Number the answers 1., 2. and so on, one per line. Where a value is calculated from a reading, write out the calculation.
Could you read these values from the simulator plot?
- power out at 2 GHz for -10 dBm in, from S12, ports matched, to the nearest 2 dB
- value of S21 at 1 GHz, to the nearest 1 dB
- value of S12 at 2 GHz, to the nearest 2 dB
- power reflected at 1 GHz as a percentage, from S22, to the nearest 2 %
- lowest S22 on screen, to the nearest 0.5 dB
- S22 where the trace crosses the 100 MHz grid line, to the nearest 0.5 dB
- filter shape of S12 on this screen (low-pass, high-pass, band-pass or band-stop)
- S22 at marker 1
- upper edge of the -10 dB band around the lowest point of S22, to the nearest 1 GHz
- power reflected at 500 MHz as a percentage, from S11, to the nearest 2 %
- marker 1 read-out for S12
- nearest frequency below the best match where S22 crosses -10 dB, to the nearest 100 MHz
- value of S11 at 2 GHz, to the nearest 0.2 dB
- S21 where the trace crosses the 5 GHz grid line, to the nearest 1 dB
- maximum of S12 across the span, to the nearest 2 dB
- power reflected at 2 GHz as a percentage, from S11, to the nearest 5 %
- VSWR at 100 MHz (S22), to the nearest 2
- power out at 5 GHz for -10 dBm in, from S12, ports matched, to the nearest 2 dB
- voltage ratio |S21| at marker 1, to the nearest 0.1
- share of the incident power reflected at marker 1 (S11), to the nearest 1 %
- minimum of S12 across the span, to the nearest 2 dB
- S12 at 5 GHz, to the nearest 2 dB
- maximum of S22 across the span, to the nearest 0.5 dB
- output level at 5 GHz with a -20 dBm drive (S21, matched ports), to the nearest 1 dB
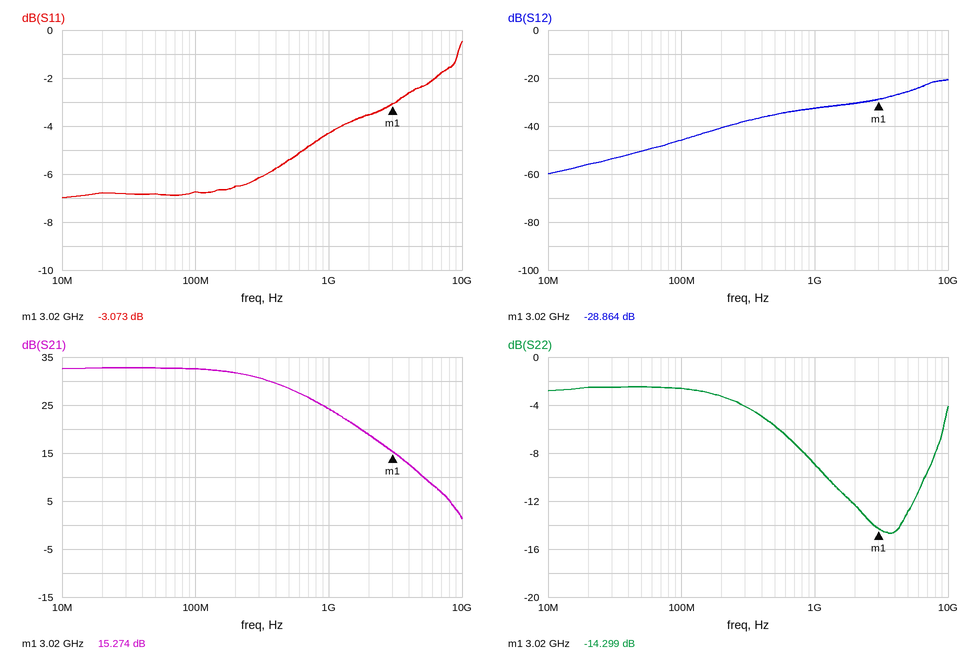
1. -10 dBm + (-30 dB) = -40 dBm
2. 24 dB
3. -30 dB
4. 10^(-9/10) ≈ 12.6 %, so 12 % to the nearest 2 %
5. -14.5 dB
6. -2.5 dB
7. high-pass
8. -14.299 dB
9. 7 GHz
10. 10^(-5.4/10) ≈ 28.8 %, so 28 % to the nearest 2 %
11. -28.864 dB
12. 1.2 GHz
13. -3.6 dB
14. 10 dB
15. -20 dB
16. 10^(-3.6/10) ≈ 43.7 %, so 45 % to the nearest 5 %
17. |Γ| = 10^(-2.5/20) = 0.7499; VSWR = (1 + 0.7499)/(1 − 0.7499) ≈ 7.00, so 6 to the nearest 2
18. -10 dBm + (-26 dB) = -36 dBm
19. 10^(15.274/20) ≈ 5.8
20. 10^(-3.073/10) ≈ 49 %
21. -60 dB
22. -26 dB
23. -2.5 dB
24. -20 dBm + (10 dB) = -10 dBm
